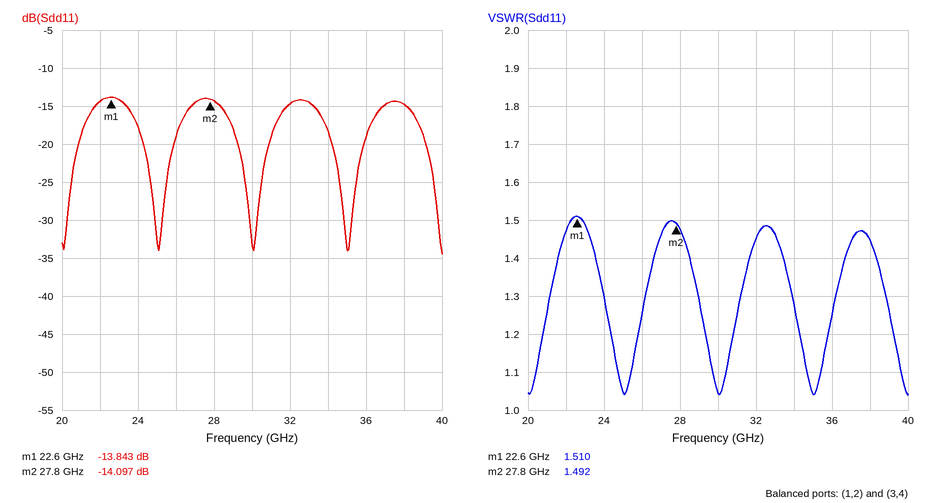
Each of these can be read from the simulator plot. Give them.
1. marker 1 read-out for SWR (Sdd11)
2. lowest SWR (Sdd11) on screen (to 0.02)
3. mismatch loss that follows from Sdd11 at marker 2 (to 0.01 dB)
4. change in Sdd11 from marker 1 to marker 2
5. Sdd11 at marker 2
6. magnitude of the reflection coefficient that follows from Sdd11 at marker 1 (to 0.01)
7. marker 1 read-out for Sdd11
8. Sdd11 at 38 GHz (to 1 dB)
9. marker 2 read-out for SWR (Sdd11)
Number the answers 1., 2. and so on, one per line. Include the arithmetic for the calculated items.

1. 1.510
2. 1.04
3. −10 log10(1 − 10^(-14.097/10)) ≈ 0.17 dB
4. -14.097 − (-13.843) = -0.254 dB
5. -14.097 dB
6. 10^(-13.843/20) ≈ 0.20
7. -13.843 dB
8. -15 dB
9. 1.492
